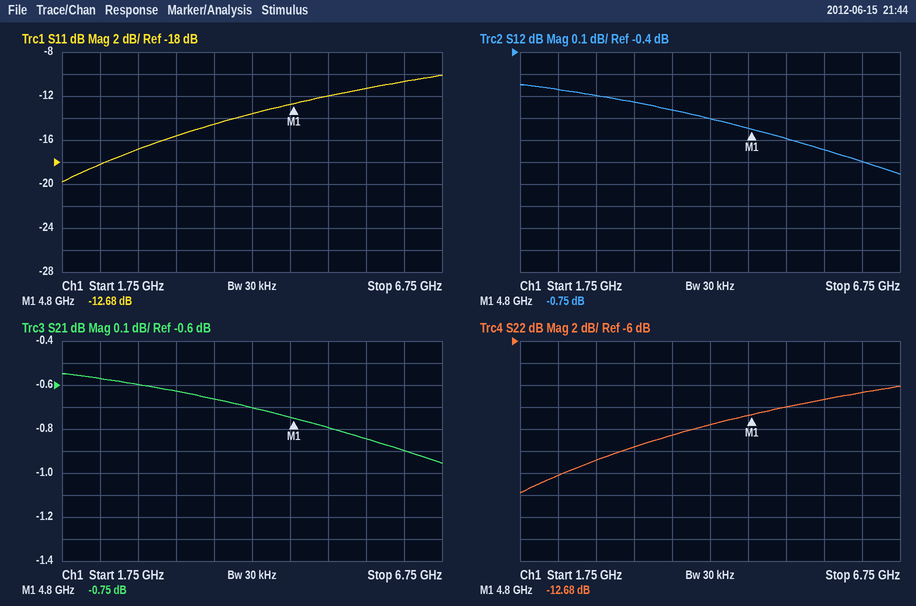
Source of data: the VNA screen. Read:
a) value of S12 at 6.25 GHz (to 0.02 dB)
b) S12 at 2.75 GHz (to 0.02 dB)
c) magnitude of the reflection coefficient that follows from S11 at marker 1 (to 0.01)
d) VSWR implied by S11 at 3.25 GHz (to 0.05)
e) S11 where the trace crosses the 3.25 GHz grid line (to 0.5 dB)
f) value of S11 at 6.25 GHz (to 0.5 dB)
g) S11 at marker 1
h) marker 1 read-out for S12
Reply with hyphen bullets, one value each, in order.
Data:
- -0.90 dB
- -0.60 dB
- 0.23
- 1.40
- -15.5 dB
- -10.5 dB
- -12.68 dB
- -0.75 dB
